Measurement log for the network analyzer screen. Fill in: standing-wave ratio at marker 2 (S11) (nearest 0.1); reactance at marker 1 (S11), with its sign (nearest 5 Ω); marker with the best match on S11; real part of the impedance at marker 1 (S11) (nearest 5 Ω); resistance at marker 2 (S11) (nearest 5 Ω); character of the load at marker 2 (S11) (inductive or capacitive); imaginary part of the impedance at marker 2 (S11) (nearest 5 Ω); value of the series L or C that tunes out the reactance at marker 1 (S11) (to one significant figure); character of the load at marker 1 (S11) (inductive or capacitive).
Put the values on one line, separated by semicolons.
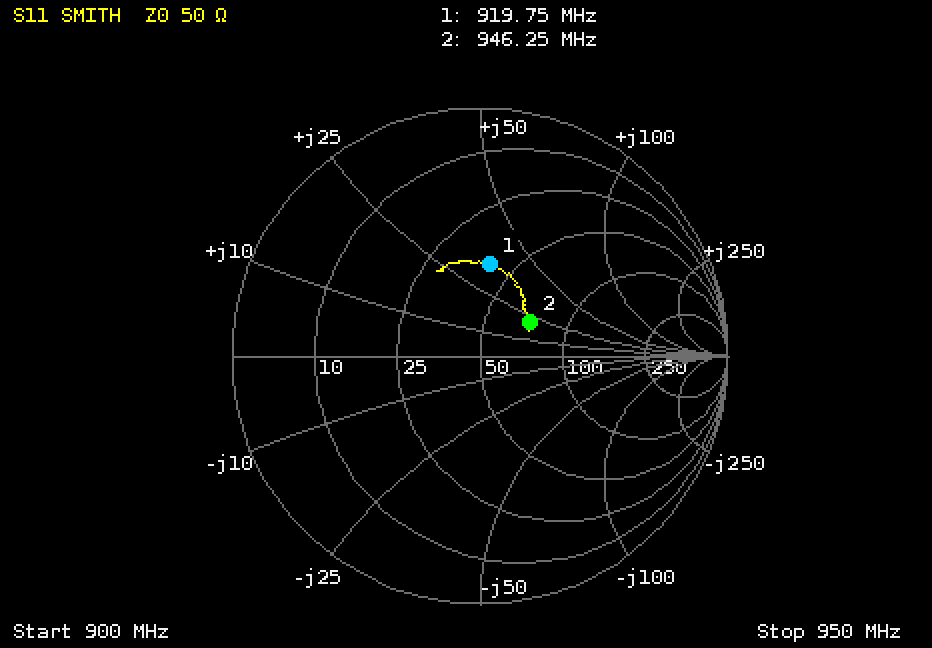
1.6; +35 Ω; marker 2; 40 Ω; 70 Ω; inductive; +20 Ω; 5 pF; inductive
